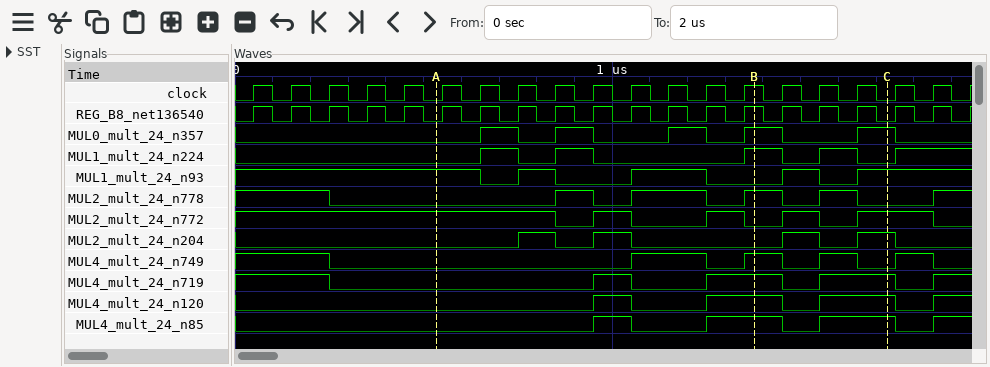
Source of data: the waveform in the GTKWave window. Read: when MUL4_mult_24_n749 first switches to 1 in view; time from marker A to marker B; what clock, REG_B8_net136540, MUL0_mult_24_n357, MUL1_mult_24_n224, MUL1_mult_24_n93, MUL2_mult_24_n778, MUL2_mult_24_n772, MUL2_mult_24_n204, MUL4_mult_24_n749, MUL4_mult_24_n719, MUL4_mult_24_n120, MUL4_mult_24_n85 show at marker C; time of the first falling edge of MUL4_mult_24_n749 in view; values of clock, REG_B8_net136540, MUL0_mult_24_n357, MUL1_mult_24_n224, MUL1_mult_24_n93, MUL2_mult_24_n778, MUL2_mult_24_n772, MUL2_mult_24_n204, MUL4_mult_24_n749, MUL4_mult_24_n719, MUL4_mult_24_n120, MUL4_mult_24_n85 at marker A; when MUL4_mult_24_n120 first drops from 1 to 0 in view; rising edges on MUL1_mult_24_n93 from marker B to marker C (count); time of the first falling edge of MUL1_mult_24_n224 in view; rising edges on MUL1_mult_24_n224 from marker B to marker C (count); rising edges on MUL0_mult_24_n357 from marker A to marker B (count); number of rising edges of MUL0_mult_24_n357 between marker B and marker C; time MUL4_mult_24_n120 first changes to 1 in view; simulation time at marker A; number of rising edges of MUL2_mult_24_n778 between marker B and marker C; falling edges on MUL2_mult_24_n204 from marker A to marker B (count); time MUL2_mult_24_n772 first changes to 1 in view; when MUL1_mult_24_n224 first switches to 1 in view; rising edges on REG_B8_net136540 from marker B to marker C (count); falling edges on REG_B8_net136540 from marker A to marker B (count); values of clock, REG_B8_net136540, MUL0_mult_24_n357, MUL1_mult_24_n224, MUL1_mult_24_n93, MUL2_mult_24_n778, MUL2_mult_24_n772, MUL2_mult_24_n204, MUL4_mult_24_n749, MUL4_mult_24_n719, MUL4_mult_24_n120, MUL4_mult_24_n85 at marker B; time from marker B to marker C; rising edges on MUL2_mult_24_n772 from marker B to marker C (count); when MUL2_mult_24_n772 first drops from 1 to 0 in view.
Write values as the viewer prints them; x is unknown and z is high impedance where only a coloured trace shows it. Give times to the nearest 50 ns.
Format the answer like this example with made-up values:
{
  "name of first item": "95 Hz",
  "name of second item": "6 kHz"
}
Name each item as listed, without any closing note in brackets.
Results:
{
  "when MUL4_mult_24_n749 first switches to 1 in view": "1050 ns",
  "time from marker A to marker B": "850 ns",
  "what clock, REG_B8_net136540, MUL0_mult_24_n357, MUL1_mult_24_n224, MUL1_mult_24_n93, MUL2_mult_24_n778, MUL2_mult_24_n772, MUL2_mult_24_n204, MUL4_mult_24_n749, MUL4_mult_24_n719, MUL4_mult_24_n120, MUL4_mult_24_n85 show at marker C": "clock=0, REG_B8_net136540=0, MUL0_mult_24_n357=1, MUL1_mult_24_n224=0, MUL1_mult_24_n93=1, MUL2_mult_24_n778=0, MUL2_mult_24_n772=1, MUL2_mult_24_n204=1, MUL4_mult_24_n749=0, MUL4_mult_24_n719=1, MUL4_mult_24_n120=1, MUL4_mult_24_n85=1",
  "time of the first falling edge of MUL4_mult_24_n749 in view": "250 ns",
  "values of clock, REG_B8_net136540, MUL0_mult_24_n357, MUL1_mult_24_n224, MUL1_mult_24_n93, MUL2_mult_24_n778, MUL2_mult_24_n772, MUL2_mult_24_n204, MUL4_mult_24_n749, MUL4_mult_24_n719, MUL4_mult_24_n120, MUL4_mult_24_n85 at marker A": "clock=0, REG_B8_net136540=0, MUL0_mult_24_n357=0, MUL1_mult_24_n224=0, MUL1_mult_24_n93=1, MUL2_mult_24_n778=0, MUL2_mult_24_n772=1, MUL2_mult_24_n204=0, MUL4_mult_24_n749=0, MUL4_mult_24_n719=0, MUL4_mult_24_n120=0, MUL4_mult_24_n85=0",
  "when MUL4_mult_24_n120 first drops from 1 to 0 in view": "1050 ns",
  "rising edges on MUL1_mult_24_n93 from marker B to marker C": "2",
  "time of the first falling edge of MUL1_mult_24_n224 in view": "750 ns",
  "rising edges on MUL1_mult_24_n224 from marker B to marker C": "1",
  "rising edges on MUL0_mult_24_n357 from marker A to marker B": "4",
  "number of rising edges of MUL0_mult_24_n357 between marker B and marker C": "1",
  "time MUL4_mult_24_n120 first changes to 1 in view": "950 ns",
  "simulation time at marker A": "550 ns",
  "number of rising edges of MUL2_mult_24_n778 between marker B and marker C": "1",
  "falling edges on MUL2_mult_24_n204 from marker A to marker B": "2",
  "time MUL2_mult_24_n772 first changes to 1 in view": "950 ns",
  "when MUL1_mult_24_n224 first switches to 1 in view": "650 ns",
  "rising edges on REG_B8_net136540 from marker B to marker C": "3",
  "falling edges on REG_B8_net136540 from marker A to marker B": "8",
  "values of clock, REG_B8_net136540, MUL0_mult_24_n357, MUL1_mult_24_n224, MUL1_mult_24_n93, MUL2_mult_24_n778, MUL2_mult_24_n772, MUL2_mult_24_n204, MUL4_mult_24_n749, MUL4_mult_24_n719, MUL4_mult_24_n120, MUL4_mult_24_n85 at marker B": "clock=1, REG_B8_net136540=1, MUL0_mult_24_n357=1, MUL1_mult_24_n224=1, MUL1_mult_24_n93=0, MUL2_mult_24_n778=1, MUL2_mult_24_n772=0, MUL2_mult_24_n204=0, MUL4_mult_24_n749=1, MUL4_mult_24_n719=1, MUL4_mult_24_n120=1, MUL4_mult_24_n85=1",
  "time from marker B to marker C": "350 ns",
  "rising edges on MUL2_mult_24_n772 from marker B to marker C": "2",
  "when MUL2_mult_24_n772 first drops from 1 to 0 in view": "850 ns"
}
